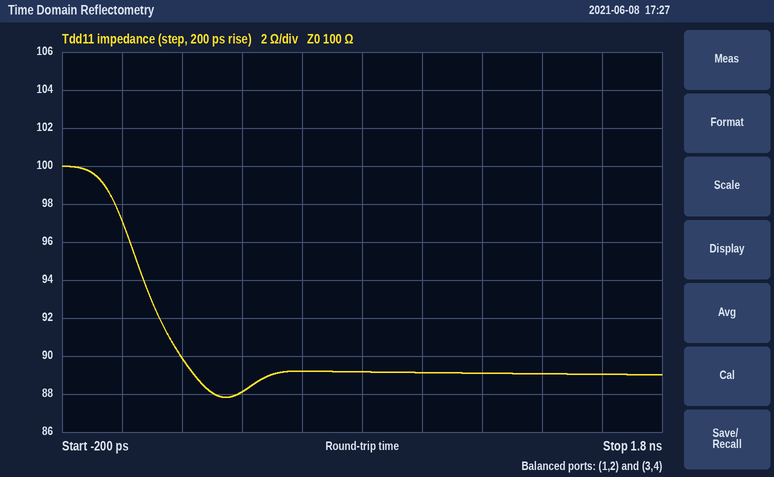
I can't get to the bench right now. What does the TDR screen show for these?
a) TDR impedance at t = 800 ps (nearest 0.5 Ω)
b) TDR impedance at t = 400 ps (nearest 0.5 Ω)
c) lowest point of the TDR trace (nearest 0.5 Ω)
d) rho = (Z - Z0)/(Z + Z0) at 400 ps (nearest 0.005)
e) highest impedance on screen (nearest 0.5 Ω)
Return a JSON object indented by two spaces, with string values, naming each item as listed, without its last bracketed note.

{
  "TDR impedance at t = 800 ps": "89.0 Ω",
  "TDR impedance at t = 400 ps": "88.0 Ω",
  "lowest point of the TDR trace": "88.0 Ω",
  "rho = (Z - Z0)/(Z + Z0) at 400 ps": "-0.065",
  "highest impedance on screen": "100.0 Ω"
}
